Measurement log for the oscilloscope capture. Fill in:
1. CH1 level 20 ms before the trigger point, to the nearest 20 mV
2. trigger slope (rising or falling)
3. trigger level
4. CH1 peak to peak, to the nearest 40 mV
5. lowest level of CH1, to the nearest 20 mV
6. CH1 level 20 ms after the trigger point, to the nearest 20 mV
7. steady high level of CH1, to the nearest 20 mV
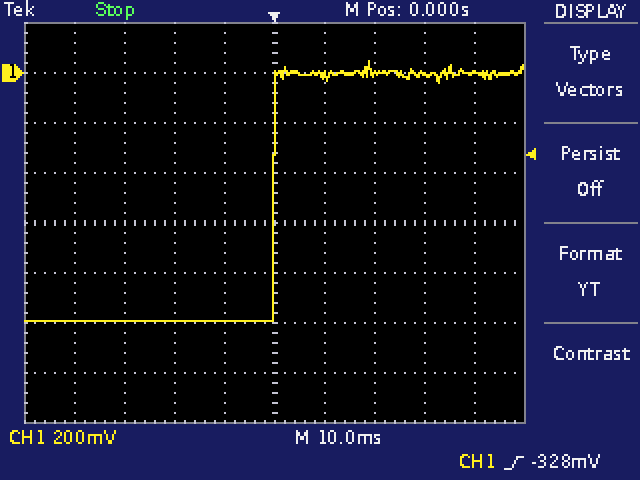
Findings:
-1.00 V
rising
-328 mV
1.04 V
-1.00 V
0 mV
0 mV
